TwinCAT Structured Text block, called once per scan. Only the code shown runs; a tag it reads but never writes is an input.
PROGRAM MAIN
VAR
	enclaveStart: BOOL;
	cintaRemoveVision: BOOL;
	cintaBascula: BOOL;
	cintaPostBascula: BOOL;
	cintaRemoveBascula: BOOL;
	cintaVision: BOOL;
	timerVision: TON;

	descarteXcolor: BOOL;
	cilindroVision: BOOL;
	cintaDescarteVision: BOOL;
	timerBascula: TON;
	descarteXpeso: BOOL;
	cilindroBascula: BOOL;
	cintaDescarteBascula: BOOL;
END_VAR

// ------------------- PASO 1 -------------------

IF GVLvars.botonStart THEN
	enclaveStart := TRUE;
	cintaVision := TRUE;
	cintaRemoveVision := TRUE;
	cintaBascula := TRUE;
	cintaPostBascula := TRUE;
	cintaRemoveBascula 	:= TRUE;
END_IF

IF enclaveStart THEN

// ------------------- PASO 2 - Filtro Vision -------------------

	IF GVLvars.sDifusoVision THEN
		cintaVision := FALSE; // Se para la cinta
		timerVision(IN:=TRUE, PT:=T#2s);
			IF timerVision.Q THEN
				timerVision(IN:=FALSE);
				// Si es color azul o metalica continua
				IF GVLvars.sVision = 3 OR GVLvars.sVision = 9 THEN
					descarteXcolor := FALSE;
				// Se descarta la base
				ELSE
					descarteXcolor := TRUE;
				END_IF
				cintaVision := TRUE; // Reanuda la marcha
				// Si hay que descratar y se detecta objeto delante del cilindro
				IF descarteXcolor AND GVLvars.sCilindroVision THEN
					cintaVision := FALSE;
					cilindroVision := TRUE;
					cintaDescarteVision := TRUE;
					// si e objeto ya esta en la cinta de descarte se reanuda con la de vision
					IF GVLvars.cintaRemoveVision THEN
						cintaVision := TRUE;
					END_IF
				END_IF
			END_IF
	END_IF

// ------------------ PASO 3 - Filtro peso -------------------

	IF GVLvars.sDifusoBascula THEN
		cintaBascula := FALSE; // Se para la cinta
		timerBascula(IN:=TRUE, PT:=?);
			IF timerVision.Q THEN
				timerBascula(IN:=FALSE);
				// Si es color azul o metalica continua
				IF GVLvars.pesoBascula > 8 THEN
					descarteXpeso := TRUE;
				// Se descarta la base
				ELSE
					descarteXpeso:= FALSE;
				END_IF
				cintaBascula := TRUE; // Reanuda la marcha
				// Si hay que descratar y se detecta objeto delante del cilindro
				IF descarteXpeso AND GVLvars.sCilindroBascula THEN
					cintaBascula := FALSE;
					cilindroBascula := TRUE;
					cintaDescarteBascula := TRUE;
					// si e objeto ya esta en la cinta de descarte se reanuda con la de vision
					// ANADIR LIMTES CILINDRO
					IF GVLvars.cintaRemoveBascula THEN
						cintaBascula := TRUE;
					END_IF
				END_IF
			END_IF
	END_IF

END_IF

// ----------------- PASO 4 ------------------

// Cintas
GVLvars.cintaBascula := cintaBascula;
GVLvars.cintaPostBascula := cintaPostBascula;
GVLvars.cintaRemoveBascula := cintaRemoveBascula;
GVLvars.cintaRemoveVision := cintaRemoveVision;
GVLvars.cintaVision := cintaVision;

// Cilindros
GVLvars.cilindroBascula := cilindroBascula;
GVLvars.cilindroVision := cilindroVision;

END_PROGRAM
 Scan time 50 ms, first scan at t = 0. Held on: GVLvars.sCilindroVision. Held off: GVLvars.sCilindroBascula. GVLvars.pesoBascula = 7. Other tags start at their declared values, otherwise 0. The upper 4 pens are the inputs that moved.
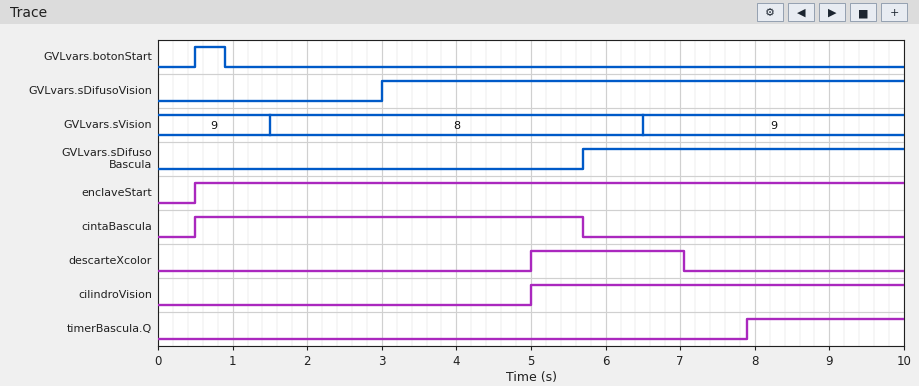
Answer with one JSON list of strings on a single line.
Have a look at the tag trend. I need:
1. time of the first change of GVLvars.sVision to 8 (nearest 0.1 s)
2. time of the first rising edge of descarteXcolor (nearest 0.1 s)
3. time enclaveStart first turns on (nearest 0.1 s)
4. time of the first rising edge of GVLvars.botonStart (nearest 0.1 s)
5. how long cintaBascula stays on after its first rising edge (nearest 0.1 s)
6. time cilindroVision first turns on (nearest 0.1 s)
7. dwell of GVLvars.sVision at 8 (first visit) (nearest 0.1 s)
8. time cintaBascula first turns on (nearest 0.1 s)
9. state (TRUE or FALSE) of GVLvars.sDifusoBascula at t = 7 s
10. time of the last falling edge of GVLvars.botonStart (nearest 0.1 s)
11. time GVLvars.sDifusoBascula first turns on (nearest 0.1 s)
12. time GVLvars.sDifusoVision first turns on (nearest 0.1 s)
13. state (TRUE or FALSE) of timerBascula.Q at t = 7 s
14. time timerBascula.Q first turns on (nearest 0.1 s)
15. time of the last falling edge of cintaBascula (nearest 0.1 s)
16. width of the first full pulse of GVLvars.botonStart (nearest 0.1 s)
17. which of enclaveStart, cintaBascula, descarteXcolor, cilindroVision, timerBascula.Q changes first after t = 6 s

["1.5 s", "5.0 s", "0.5 s", "0.5 s", "5.2 s", "5.0 s", "5.0 s", "0.5 s", "TRUE", "0.9 s", "5.7 s", "3.0 s", "FALSE", "7.9 s", "5.7 s", "0.4 s", "descarteXcolor"]
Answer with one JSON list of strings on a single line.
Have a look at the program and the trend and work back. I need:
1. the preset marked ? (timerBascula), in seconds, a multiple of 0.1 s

["2.2 s"]
